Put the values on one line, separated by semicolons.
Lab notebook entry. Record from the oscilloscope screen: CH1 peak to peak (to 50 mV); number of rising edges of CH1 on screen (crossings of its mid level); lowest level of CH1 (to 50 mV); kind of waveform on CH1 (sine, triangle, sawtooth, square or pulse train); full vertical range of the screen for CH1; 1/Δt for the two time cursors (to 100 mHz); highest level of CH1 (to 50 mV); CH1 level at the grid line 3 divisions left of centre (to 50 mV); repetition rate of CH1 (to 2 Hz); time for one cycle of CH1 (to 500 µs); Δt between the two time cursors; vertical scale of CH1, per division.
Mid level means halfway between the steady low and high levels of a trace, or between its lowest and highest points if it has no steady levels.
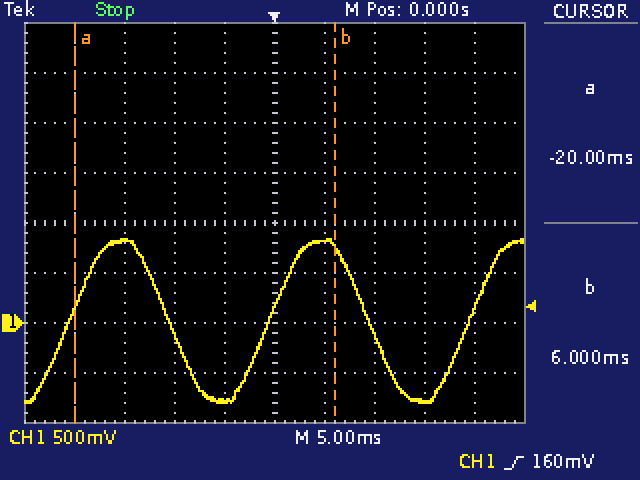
1.65 V; 3; -800 mV; sine; 4 V; 38.5 Hz; 850 mV; 800 mV; 50 Hz; 20.0 ms; 26.0 ms; 500 mV
